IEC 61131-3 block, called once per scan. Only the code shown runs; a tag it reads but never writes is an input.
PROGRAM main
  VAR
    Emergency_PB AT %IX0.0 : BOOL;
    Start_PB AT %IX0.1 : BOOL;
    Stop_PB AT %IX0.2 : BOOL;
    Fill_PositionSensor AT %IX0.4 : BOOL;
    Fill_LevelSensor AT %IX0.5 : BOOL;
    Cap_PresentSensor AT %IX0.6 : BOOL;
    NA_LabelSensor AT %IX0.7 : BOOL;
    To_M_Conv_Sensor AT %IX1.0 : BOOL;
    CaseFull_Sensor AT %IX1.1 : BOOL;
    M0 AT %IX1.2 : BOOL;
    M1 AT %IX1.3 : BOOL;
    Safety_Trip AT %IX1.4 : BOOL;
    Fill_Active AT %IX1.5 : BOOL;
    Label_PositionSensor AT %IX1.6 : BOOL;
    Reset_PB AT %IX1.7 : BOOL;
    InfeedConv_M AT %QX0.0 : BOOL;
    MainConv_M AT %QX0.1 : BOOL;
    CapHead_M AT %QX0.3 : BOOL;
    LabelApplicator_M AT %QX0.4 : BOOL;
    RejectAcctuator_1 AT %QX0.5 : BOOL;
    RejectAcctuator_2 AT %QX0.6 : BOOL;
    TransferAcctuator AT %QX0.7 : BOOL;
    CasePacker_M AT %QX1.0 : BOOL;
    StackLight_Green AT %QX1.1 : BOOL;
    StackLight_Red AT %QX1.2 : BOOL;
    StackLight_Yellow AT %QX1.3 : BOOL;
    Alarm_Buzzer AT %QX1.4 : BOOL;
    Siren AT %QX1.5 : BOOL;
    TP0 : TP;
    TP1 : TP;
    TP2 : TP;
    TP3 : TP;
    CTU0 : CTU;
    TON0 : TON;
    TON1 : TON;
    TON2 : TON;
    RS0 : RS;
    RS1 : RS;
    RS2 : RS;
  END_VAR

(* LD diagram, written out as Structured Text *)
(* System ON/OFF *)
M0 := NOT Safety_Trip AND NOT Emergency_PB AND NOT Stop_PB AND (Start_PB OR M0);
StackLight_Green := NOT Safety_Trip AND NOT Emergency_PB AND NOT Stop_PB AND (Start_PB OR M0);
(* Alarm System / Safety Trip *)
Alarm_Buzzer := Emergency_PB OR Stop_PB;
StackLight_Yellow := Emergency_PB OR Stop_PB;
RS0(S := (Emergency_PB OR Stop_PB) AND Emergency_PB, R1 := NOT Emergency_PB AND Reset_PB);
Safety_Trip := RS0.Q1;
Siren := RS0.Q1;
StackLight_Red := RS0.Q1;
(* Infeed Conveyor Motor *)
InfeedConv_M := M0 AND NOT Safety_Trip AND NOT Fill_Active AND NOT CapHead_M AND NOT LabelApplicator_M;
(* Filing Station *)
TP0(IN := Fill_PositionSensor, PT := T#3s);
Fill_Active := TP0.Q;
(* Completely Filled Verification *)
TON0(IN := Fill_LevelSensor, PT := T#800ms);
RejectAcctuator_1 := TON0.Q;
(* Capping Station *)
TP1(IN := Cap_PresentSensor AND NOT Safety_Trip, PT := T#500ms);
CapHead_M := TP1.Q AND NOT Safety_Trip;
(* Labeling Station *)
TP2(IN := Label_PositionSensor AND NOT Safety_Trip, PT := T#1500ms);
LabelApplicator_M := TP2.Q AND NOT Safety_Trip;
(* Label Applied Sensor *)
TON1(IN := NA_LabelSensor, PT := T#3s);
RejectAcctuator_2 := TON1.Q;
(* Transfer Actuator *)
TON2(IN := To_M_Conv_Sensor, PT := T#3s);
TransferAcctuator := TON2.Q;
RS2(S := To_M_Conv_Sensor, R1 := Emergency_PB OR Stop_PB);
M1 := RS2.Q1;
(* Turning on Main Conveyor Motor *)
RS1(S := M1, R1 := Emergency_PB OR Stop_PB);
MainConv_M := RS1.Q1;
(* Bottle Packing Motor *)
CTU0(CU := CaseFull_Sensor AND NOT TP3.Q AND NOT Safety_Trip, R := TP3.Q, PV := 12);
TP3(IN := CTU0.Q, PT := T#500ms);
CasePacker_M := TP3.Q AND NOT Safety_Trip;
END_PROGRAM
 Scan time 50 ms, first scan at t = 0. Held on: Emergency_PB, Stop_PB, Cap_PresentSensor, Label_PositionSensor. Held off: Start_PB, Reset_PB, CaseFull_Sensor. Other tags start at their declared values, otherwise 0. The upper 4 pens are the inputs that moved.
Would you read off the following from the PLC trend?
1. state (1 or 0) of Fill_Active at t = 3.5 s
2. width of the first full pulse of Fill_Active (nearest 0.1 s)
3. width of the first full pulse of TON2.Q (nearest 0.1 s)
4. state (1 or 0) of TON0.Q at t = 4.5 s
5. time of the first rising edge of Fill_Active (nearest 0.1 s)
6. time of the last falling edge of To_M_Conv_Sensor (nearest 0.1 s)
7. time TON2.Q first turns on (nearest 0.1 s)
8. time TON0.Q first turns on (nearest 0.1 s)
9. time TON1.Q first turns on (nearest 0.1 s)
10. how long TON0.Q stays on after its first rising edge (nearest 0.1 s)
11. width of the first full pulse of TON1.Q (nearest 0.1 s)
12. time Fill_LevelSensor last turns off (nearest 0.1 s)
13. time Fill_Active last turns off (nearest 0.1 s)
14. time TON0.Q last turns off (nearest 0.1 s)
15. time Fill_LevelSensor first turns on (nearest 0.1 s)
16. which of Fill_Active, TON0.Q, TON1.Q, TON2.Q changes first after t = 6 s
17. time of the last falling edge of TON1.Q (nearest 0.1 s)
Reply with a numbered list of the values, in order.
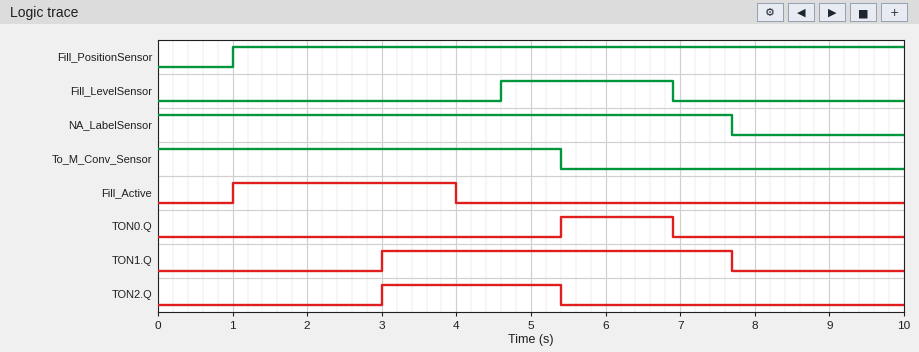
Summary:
1. 1
2. 3.0 s
3. 2.4 s
4. 0
5. 1.0 s
6. 5.4 s
7. 3.0 s
8. 5.4 s
9. 3.0 s
10. 1.5 s
11. 4.7 s
12. 6.9 s
13. 4.0 s
14. 6.9 s
15. 4.6 s
16. TON0.Q
17. 7.7 s
